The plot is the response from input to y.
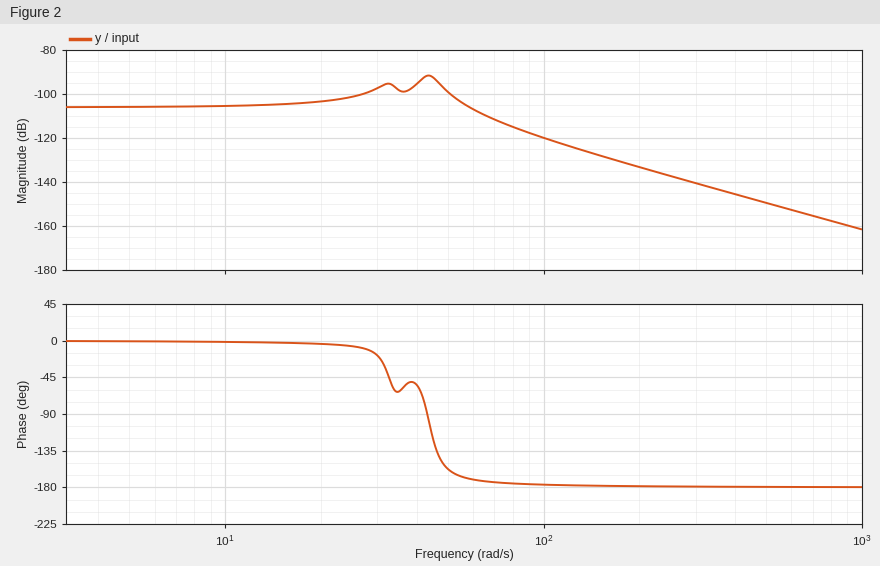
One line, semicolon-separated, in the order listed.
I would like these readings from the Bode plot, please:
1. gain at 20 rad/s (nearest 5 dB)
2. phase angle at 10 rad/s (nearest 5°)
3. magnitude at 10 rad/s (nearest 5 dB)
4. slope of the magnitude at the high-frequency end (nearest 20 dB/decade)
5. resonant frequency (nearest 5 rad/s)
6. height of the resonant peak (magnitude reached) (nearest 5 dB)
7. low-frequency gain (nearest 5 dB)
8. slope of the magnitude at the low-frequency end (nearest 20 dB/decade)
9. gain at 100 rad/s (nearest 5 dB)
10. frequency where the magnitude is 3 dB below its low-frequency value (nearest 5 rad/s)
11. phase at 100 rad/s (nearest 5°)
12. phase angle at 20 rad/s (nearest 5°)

-105 dB; 0°; -105 dB; -40 dB/decade; 45 rad/s; -90 dB; -105 dB; 0 dB/decade; -120 dB; 65 rad/s; -175°; -5°
